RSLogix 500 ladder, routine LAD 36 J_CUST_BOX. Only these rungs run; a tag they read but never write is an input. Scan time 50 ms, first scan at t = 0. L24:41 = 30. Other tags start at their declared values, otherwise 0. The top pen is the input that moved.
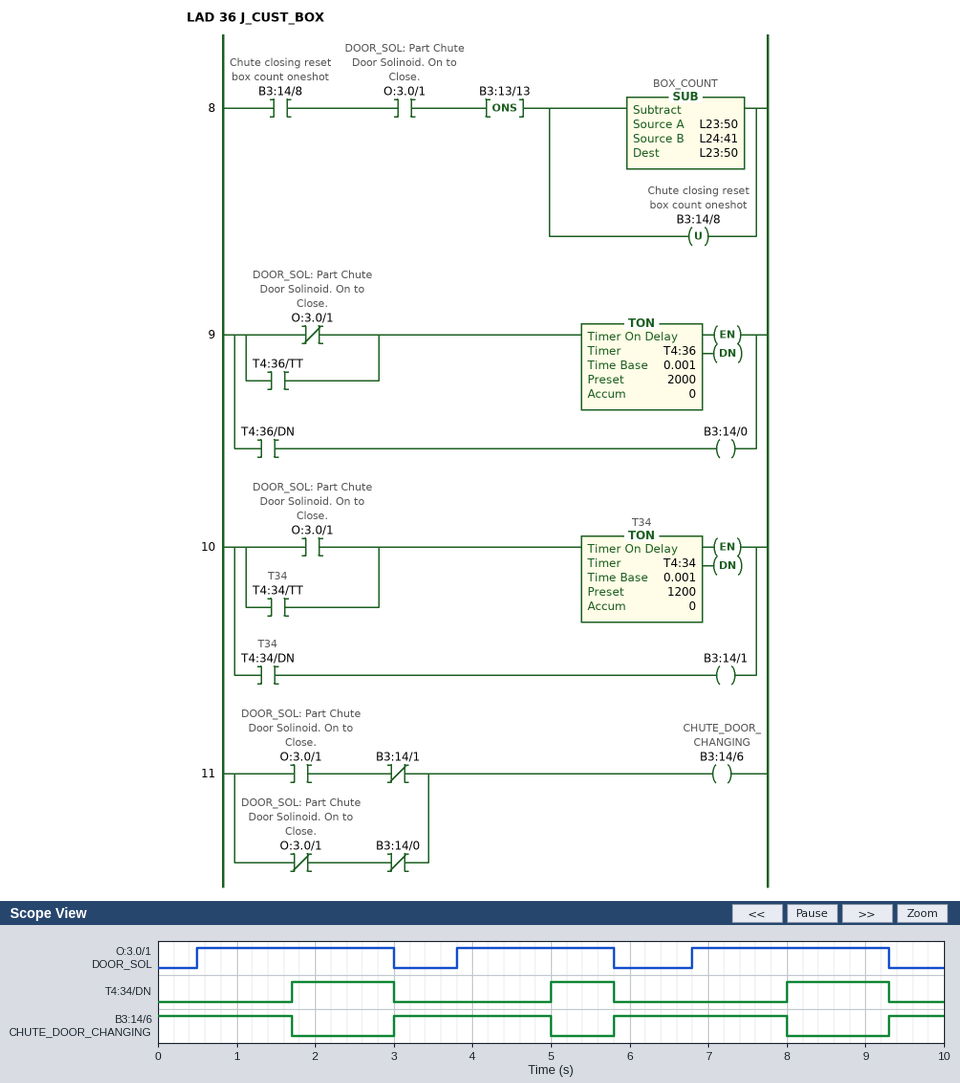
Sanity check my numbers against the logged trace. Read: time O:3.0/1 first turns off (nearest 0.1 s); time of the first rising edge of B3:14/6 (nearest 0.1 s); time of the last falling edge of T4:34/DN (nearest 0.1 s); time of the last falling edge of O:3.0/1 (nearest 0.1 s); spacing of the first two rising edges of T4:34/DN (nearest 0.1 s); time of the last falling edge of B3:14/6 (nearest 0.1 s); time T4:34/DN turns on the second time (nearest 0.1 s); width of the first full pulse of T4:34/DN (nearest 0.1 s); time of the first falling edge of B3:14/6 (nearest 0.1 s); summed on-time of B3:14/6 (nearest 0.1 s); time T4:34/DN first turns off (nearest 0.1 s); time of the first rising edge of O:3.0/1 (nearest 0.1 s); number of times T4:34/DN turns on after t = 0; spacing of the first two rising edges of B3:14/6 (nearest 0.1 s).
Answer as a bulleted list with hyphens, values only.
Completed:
- 3.0 s
- 3.0 s
- 9.3 s
- 9.3 s
- 3.3 s
- 8.0 s
- 5.0 s
- 1.3 s
- 1.7 s
- 6.6 s
- 3.0 s
- 0.5 s
- 3
- 2.8 s
